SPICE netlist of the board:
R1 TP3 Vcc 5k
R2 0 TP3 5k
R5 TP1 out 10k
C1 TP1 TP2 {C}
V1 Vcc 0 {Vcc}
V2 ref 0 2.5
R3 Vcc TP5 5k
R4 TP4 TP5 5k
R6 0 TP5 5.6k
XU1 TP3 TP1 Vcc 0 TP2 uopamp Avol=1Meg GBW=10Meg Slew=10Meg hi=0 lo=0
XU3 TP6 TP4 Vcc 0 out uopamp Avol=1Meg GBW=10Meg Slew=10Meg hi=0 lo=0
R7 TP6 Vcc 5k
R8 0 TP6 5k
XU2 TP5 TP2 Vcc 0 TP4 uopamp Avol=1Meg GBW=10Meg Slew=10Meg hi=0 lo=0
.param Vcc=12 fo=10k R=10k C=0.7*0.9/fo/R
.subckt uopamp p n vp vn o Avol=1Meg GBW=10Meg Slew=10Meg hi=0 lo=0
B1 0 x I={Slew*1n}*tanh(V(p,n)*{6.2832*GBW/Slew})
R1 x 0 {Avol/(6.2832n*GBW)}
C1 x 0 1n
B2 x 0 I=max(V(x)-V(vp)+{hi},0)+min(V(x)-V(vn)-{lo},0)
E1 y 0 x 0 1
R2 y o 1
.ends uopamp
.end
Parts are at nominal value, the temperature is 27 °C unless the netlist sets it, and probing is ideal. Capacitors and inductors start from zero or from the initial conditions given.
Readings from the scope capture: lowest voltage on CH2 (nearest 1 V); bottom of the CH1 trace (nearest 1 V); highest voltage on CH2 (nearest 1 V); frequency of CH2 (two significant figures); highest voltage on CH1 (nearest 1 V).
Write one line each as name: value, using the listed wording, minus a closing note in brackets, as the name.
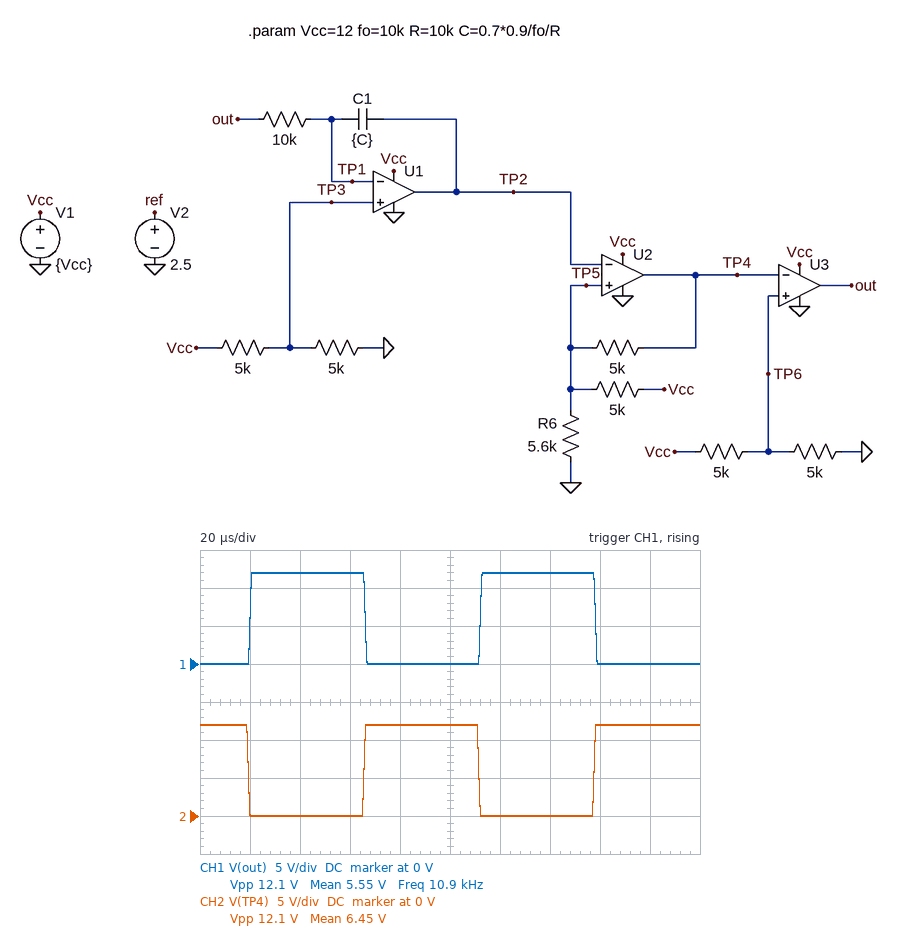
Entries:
lowest voltage on CH2: 0 V
bottom of the CH1 trace: 0 V
highest voltage on CH2: 12 V
frequency of CH2: 11 kHz
highest voltage on CH1: 12 V
